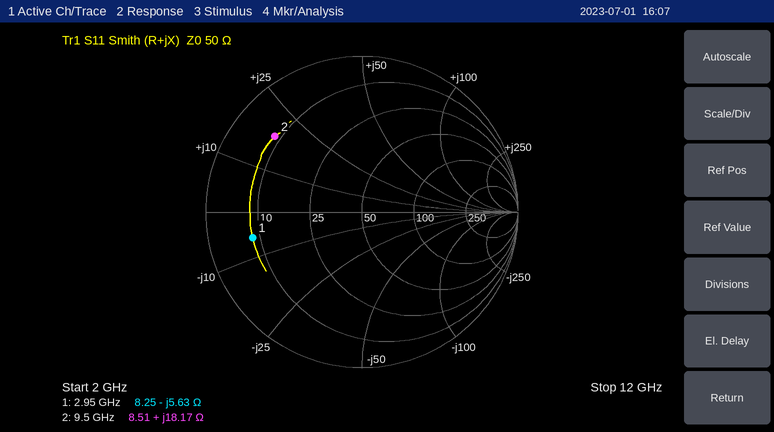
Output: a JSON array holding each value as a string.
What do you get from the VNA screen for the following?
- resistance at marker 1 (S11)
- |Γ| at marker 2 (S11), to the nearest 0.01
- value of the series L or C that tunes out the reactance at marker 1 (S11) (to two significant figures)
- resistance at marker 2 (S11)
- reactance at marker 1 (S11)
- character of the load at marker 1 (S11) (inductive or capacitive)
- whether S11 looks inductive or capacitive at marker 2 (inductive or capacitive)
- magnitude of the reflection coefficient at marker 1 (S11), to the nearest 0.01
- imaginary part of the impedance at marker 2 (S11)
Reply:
["8.25 Ω", "0.74", "300 pH", "8.51 Ω", "-5.63 Ω", "capacitive", "inductive", "0.72", "+18.17 Ω"]
